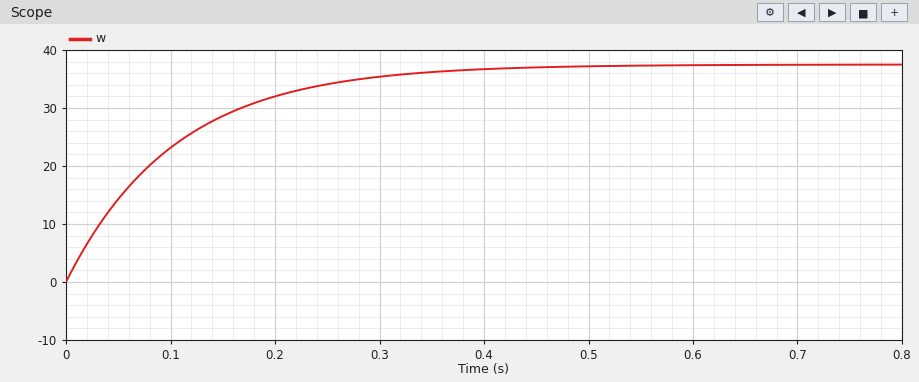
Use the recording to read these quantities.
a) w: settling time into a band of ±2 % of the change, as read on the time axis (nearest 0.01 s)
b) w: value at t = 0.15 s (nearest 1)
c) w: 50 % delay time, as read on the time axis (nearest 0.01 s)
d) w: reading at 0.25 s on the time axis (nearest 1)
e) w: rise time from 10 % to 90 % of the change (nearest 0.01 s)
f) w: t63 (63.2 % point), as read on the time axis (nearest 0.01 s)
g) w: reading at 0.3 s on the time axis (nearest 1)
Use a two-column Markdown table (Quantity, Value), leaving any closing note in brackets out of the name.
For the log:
| Quantity | Value |
|---|---|
| w: settling time into a band of ±2 % of the change, as read on the time axis | 0.41 s |
| w: value at t = 0.15 s | 29 |
| w: 50 % delay time, as read on the time axis | 0.07 s |
| w: reading at 0.25 s on the time axis | 34 |
| w: rise time from 10 % to 90 % of the change | 0.23 s |
| w: t63 (63.2 % point), as read on the time axis | 0.10 s |
| w: reading at 0.3 s on the time axis | 35 |
